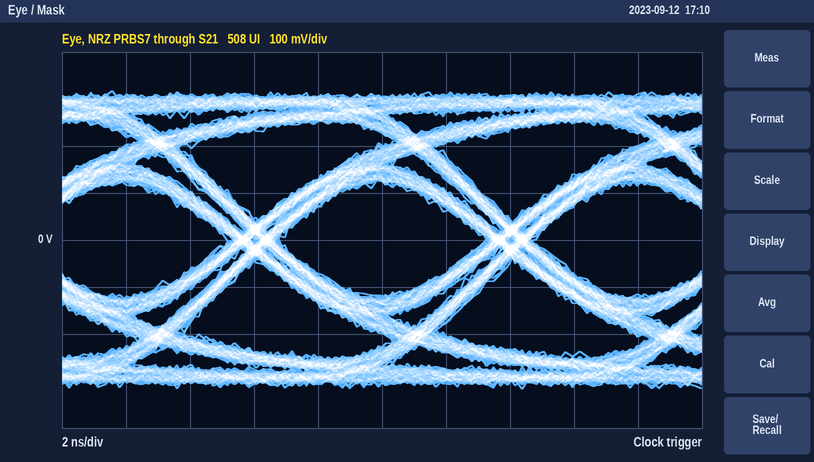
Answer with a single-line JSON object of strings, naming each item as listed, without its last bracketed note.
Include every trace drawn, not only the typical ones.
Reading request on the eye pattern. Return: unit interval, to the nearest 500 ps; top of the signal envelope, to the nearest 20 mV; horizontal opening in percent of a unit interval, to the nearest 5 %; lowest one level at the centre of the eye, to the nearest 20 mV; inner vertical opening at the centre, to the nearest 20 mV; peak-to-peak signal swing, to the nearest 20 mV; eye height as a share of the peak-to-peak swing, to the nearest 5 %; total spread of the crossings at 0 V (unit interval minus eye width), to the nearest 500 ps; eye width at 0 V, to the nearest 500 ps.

{"unit interval, to the nearest 500 ps": "8.0 ns", "top of the signal envelope, to the nearest 20 mV": "320 mV", "horizontal opening in percent of a unit interval, to the nearest 5 %": "80 %", "lowest one level at the centre of the eye, to the nearest 20 mV": "120 mV", "inner vertical opening at the centre, to the nearest 20 mV": "240 mV", "peak-to-peak signal swing, to the nearest 20 mV": "640 mV", "eye height as a share of the peak-to-peak swing, to the nearest 5 %": "40 %", "total spread of the crossings at 0 V (unit interval minus eye width), to the nearest 500 ps": "1.5 ns", "eye width at 0 V, to the nearest 500 ps": "6.5 ns"}
